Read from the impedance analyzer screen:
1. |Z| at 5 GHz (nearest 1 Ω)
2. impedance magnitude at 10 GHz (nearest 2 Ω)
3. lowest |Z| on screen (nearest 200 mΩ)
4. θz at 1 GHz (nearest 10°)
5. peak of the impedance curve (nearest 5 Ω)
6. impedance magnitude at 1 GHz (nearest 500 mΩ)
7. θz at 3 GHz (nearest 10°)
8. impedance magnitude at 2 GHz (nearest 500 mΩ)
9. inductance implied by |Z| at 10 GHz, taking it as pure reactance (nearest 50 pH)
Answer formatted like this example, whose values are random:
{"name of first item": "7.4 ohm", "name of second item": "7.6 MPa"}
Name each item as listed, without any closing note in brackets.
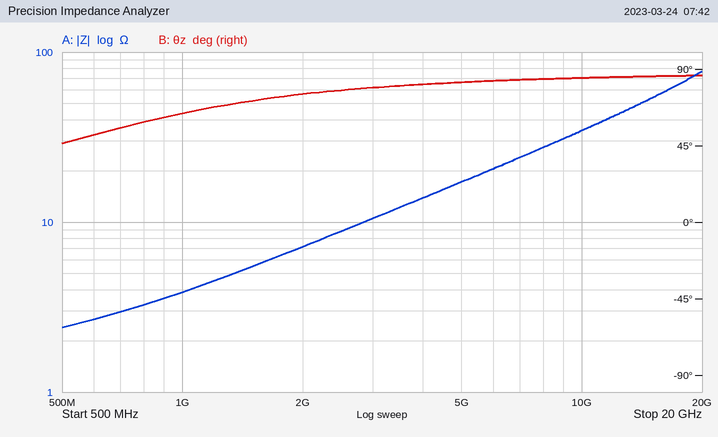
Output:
{"|Z| at 5 GHz": "17 Ω", "impedance magnitude at 10 GHz": "34 Ω", "lowest |Z| on screen": "2.4 Ω", "θz at 1 GHz": "60°", "peak of the impedance curve": "75 Ω", "impedance magnitude at 1 GHz": "4.0 Ω", "θz at 3 GHz": "80°", "impedance magnitude at 2 GHz": "7.0 Ω", "inductance implied by |Z| at 10 GHz, taking it as pure reactance": "550 pH"}
